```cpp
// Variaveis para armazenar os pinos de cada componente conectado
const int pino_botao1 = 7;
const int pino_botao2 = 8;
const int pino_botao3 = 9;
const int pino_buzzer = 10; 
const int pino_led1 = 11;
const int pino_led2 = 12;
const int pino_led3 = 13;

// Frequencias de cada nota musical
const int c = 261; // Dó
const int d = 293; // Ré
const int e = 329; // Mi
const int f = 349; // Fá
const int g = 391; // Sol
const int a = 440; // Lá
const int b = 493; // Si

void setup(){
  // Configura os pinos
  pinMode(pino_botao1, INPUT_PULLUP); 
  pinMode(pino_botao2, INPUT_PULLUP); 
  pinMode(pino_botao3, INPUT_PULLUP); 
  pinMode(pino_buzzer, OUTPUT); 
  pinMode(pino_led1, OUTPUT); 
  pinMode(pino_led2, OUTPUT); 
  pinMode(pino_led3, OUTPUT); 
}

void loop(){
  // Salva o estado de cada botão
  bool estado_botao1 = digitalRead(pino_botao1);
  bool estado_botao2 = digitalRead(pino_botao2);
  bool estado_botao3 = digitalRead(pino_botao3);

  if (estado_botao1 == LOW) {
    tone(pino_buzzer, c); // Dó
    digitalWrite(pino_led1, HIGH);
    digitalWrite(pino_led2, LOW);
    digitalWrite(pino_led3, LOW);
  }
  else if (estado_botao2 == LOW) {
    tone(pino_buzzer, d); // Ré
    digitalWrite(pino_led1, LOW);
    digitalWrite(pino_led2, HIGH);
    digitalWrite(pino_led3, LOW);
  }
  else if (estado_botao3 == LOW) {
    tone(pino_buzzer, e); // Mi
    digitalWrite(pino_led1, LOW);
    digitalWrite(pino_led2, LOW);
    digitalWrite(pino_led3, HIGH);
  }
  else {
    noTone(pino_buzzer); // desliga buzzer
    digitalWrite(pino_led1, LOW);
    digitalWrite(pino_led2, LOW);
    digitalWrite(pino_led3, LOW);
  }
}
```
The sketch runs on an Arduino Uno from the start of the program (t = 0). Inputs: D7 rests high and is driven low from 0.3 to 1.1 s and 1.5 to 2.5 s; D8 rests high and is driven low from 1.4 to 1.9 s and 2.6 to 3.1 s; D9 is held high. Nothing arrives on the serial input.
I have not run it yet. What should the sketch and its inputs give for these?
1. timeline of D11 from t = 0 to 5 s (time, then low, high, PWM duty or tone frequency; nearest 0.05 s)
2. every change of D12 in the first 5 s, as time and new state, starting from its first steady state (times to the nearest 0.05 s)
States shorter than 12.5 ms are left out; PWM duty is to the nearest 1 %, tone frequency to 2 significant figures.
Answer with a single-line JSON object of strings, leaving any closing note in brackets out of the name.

{"timeline of D11 from t = 0 to 5 s": "0 s low; 0.3 s high; 1.1 s low; 1.5 s high; 2.5 s low", "every change of D12 in the first 5 s, as time and new state, starting from its first steady state": "0 s low; 1.4 s high; 1.5 s low; 2.6 s high; 3.1 s low"}
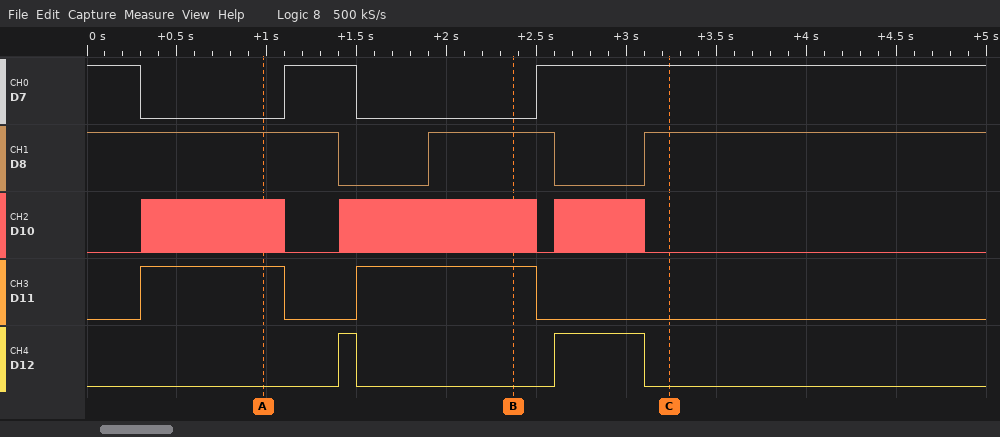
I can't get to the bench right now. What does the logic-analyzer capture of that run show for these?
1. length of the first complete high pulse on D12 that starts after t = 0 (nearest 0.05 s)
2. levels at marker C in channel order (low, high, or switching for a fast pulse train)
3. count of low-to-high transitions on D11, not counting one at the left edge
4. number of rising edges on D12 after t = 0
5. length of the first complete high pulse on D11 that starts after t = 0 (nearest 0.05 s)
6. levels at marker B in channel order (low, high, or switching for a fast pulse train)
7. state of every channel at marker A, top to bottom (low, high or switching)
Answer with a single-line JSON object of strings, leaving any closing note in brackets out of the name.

{"length of the first complete high pulse on D12 that starts after t = 0": "0.10 s", "levels at marker C in channel order": "D7 high, D8 high, D10 low, D11 low, D12 low", "count of low-to-high transitions on D11, not counting one at the left edge": "2", "number of rising edges on D12 after t = 0": "2", "length of the first complete high pulse on D11 that starts after t = 0": "0.80 s", "levels at marker B in channel order": "D7 low, D8 high, D10 switching, D11 high, D12 low", "state of every channel at marker A, top to bottom": "D7 low, D8 high, D10 switching, D11 high, D12 low"}
